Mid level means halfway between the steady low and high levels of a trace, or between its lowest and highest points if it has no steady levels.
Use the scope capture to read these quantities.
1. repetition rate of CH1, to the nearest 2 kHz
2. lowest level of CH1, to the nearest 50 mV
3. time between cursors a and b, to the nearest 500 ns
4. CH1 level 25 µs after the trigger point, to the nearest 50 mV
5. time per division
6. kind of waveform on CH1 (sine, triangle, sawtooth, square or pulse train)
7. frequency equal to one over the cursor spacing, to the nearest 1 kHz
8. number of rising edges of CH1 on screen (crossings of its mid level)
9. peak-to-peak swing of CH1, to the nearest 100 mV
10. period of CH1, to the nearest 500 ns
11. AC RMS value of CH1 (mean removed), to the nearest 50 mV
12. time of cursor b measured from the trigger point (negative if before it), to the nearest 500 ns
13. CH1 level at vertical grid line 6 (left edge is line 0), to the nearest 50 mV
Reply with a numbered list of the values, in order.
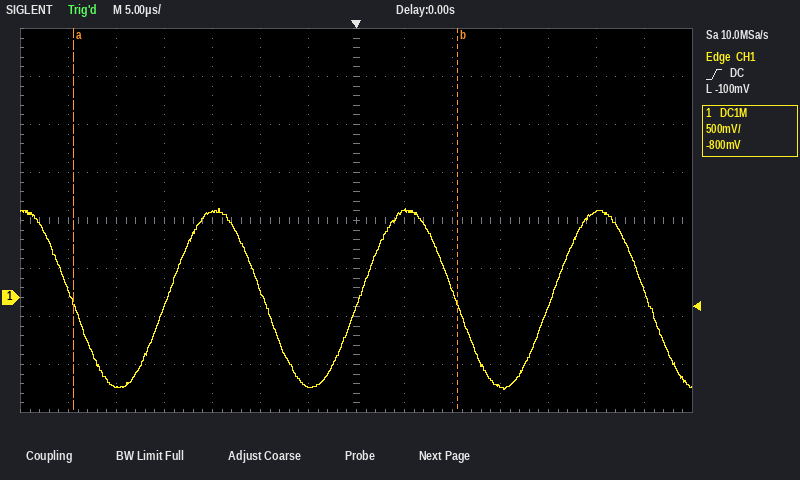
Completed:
1. 50 kHz
2. -950 mV
3. 40.0 µs
4. 900 mV
5. 5 µs
6. sine
7. 25 kHz
8. 3
9. 1.90 V
10. 20.0 µs
11. 650 mV
12. +10.5 µs
13. -950 mV
